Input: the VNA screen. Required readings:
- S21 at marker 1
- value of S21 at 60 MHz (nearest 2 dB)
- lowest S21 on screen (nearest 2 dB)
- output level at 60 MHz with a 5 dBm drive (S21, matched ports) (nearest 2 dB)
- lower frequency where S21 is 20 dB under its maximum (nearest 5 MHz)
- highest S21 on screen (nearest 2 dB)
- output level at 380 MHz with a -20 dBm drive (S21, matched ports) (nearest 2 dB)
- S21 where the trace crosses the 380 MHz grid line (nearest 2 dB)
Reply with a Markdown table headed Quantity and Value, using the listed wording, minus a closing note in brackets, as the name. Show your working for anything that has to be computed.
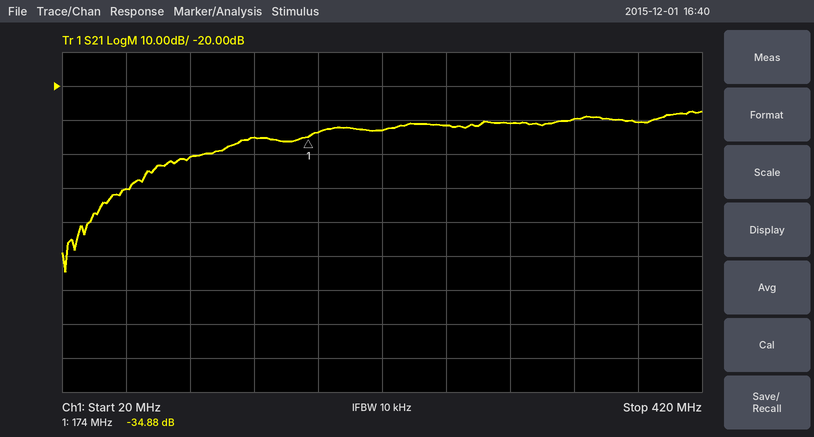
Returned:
| Quantity | Value |
|---|---|
| S21 at marker 1 | -34.88 dB |
| value of S21 at 60 MHz | -50 dB |
| lowest S21 on screen | -74 dB |
| output level at 60 MHz with a 5 dBm drive (S21, matched ports) | 5 dBm + (-50 dB) = -46 dBm |
| lower frequency where S21 is 20 dB under its maximum | 70 MHz |
| highest S21 on screen | -28 dB |
| output level at 380 MHz with a -20 dBm drive (S21, matched ports) | -20 dBm + (-30 dB) = -50 dBm |
| S21 where the trace crosses the 380 MHz grid line | -30 dB |
